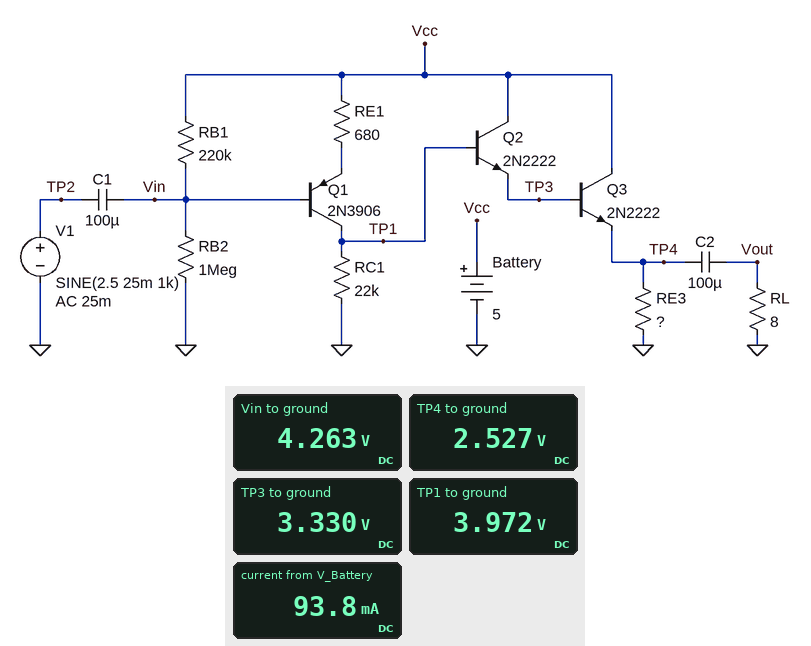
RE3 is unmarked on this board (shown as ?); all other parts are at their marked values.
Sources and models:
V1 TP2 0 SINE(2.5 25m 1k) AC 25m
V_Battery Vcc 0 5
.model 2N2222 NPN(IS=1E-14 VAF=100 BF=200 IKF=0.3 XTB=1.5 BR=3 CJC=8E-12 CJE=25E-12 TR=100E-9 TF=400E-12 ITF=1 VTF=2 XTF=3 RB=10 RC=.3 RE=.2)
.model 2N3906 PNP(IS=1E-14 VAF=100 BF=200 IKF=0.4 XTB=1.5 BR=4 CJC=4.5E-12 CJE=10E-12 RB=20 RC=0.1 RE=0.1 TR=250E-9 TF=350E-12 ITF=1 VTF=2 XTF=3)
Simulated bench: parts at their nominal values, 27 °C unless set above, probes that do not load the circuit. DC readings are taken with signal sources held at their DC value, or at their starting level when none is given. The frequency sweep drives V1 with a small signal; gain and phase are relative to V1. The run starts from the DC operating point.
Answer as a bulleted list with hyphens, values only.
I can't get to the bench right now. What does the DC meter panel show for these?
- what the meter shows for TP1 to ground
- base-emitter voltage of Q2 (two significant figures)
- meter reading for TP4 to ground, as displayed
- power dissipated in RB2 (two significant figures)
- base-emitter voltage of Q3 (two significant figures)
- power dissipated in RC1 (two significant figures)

- 3.972 V
- 640 mV
- 2.527 V
- 18 µW
- 800 mV
- 720 µW
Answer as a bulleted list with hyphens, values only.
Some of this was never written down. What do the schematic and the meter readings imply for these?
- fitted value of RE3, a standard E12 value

- 27 Ω
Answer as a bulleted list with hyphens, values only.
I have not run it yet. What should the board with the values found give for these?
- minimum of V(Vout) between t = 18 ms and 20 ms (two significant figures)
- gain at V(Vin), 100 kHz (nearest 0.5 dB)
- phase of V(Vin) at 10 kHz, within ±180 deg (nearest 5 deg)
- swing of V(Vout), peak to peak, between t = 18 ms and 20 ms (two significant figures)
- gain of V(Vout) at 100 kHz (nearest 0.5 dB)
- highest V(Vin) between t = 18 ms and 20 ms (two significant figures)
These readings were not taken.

- -480 mV
- 0 dB
- 0 deg
- 980 mV
- 26.0 dB
- 4.3 V
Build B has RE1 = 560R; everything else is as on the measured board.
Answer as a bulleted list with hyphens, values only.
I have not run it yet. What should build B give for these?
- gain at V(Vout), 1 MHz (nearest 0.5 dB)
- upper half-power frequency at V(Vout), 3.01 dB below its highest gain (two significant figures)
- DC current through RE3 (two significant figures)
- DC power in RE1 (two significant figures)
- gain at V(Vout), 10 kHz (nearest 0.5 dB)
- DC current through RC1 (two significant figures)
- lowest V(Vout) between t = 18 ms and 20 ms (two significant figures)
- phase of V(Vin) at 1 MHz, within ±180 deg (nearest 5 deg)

- 22.0 dB
- 630 kHz
- 100 mA
- 22 µW
- 27.5 dB
- 190 µA
- -550 mV
- 0 deg
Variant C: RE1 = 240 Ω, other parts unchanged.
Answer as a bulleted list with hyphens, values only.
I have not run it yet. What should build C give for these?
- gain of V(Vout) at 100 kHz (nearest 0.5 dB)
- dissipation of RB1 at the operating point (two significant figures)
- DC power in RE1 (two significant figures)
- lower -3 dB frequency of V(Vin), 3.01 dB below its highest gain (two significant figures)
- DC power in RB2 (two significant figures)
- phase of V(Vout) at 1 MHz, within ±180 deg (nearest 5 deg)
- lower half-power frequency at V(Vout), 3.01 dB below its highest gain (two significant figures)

- 31.0 dB
- 2.0 µW
- 12 µW
- 490 mHz
- 19 µW
- 110 deg
- 170 Hz
